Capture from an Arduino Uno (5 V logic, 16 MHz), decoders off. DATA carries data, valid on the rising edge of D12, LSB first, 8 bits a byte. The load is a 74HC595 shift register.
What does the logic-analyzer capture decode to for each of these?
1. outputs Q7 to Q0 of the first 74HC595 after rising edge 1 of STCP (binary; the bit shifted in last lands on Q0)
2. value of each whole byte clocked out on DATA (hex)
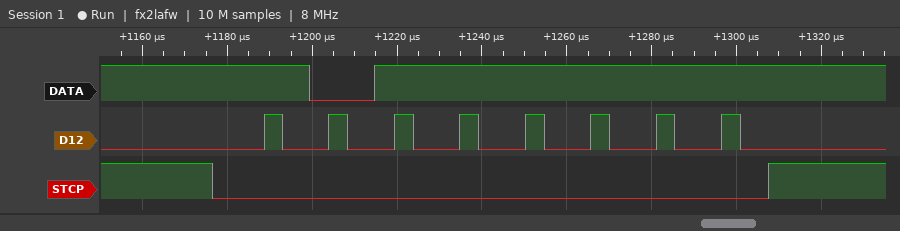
10111111
0xFD
